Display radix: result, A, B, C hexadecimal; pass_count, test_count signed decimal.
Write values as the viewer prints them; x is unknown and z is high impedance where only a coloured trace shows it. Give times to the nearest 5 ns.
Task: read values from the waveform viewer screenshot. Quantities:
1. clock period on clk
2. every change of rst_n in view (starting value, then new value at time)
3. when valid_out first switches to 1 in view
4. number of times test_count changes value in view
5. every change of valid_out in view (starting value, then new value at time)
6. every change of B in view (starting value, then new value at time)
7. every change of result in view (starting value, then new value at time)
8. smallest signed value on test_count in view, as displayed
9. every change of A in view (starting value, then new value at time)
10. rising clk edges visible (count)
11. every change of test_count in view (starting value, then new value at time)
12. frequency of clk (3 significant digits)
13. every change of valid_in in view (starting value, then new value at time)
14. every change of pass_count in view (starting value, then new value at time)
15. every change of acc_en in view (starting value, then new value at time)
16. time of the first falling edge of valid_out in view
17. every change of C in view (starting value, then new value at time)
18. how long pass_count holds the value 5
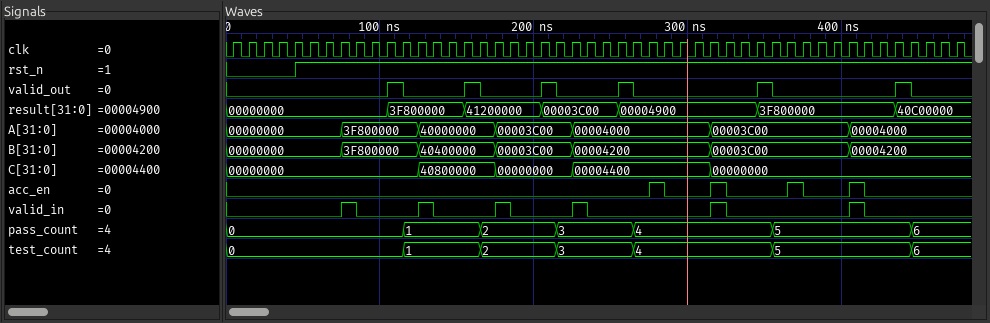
10 ns
0, 1 at 45 ns
105 ns
6
0, 1 at 105 ns, 0 at 115 ns, 1 at 155 ns, 0 at 165 ns, 1 at 205 ns, 0 at 215 ns, 1 at 255 ns, 0 at 265 ns, 1 at 345 ns, 0 at 355 ns, 1 at 435 ns, 0 at 445 ns
00000000, 3F800000 at 75 ns, 40400000 at 125 ns, 00003C00 at 175 ns, 00004200 at 225 ns, 00003C00 at 315 ns, 00004200 at 405 ns
00000000, 3F800000 at 105 ns, 41200000 at 155 ns, 00003C00 at 205 ns, 00004900 at 255 ns, 3F800000 at 345 ns, 40C00000 at 435 ns
0
00000000, 3F800000 at 75 ns, 40000000 at 125 ns, 00003C00 at 175 ns, 00004000 at 225 ns, 00003C00 at 315 ns, 00004000 at 405 ns
48
0, 1 at 115 ns, 2 at 165 ns, 3 at 215 ns, 4 at 265 ns, 5 at 355 ns, 6 at 445 ns
100 MHz
0, 1 at 75 ns, 0 at 85 ns, 1 at 125 ns, 0 at 135 ns, 1 at 175 ns, 0 at 185 ns, 1 at 225 ns, 0 at 235 ns, 1 at 315 ns, 0 at 325 ns, 1 at 405 ns, 0 at 415 ns
0, 1 at 115 ns, 2 at 165 ns, 3 at 215 ns, 4 at 265 ns, 5 at 355 ns, 6 at 445 ns
0, 1 at 275 ns, 0 at 285 ns, 1 at 315 ns, 0 at 325 ns, 1 at 365 ns, 0 at 375 ns, 1 at 405 ns, 0 at 415 ns
115 ns
00000000, 40800000 at 125 ns, 00000000 at 175 ns, 00004400 at 225 ns, 00000000 at 315 ns
90 ns
